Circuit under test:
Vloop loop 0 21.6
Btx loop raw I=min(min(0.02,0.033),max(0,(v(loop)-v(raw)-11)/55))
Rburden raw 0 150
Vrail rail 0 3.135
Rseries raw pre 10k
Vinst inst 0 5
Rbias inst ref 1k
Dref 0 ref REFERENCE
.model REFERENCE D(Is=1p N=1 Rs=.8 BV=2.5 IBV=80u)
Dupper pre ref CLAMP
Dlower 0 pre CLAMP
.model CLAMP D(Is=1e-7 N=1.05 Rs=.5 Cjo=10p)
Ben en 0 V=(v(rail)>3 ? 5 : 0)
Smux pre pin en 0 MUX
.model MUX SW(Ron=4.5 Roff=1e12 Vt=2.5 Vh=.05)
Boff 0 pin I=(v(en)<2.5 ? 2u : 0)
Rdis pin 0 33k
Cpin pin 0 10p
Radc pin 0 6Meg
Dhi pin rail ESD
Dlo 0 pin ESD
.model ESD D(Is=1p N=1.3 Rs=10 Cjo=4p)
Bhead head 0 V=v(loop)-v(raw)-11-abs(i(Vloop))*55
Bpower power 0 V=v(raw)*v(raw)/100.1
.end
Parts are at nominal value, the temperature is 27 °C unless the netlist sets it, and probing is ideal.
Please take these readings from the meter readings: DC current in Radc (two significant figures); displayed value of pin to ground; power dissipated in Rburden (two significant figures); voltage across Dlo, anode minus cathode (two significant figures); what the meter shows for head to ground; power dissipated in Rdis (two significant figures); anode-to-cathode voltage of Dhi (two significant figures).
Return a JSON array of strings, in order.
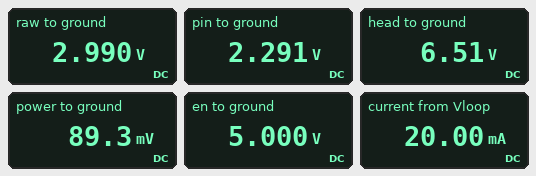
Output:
["380 nA", "2.291 V", "60 mW", "-2.3 V", "6.51 V", "160 µW", "-840 mV"]
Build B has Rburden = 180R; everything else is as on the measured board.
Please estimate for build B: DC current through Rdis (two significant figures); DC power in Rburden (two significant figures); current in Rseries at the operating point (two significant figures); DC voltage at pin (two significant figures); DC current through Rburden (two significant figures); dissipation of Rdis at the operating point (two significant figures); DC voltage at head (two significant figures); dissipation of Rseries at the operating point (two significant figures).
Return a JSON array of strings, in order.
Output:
["82 µA", "71 mW", "88 µA", "2.7 V", "20 mA", "220 µW", "5.9 V", "78 µW"]
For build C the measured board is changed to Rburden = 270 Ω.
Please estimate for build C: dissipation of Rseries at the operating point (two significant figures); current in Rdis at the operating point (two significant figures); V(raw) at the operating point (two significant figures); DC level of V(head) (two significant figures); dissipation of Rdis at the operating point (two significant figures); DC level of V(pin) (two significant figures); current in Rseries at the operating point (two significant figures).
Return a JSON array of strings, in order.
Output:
["640 µW", "85 µA", "5.3 V", "4.2 V", "240 µW", "2.8 V", "250 µA"]
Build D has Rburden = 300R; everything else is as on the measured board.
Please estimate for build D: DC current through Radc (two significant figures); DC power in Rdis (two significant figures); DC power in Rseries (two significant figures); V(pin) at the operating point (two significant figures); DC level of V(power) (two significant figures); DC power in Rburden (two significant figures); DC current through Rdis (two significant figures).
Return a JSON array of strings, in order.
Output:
["470 nA", "240 µW", "960 µW", "2.8 V", "350 mV", "120 mW", "85 µA"]
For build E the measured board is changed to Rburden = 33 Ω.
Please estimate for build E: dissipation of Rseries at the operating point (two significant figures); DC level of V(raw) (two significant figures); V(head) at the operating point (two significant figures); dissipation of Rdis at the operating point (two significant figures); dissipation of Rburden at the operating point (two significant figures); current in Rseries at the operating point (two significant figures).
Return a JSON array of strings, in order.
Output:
["2.4 µW", "660 mV", "8.8 V", "7.7 µW", "13 mW", "15 µA"]
